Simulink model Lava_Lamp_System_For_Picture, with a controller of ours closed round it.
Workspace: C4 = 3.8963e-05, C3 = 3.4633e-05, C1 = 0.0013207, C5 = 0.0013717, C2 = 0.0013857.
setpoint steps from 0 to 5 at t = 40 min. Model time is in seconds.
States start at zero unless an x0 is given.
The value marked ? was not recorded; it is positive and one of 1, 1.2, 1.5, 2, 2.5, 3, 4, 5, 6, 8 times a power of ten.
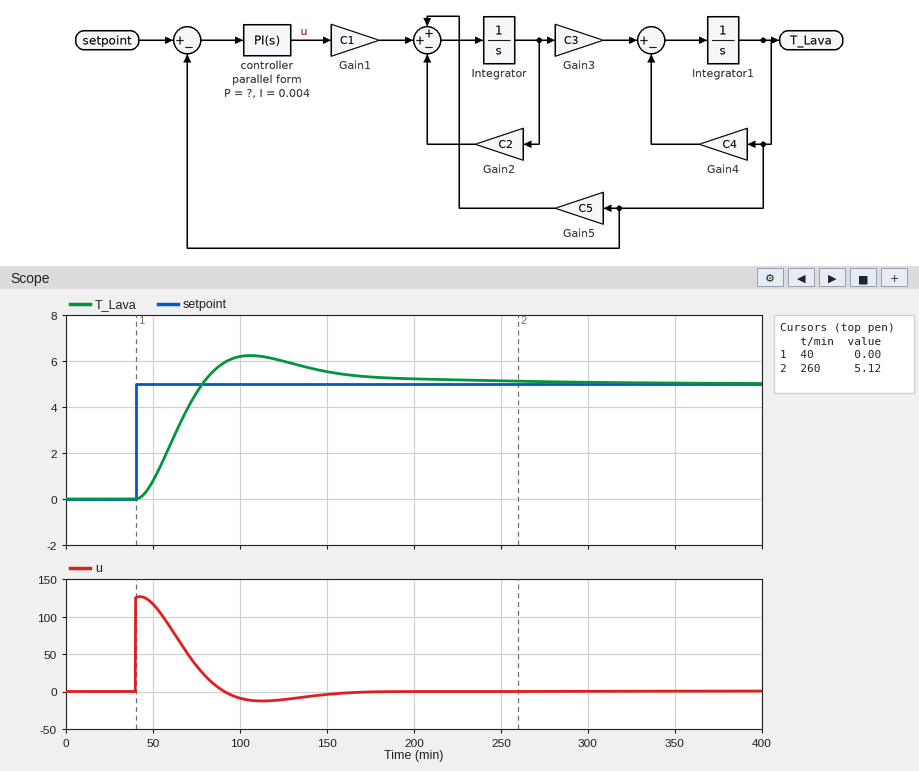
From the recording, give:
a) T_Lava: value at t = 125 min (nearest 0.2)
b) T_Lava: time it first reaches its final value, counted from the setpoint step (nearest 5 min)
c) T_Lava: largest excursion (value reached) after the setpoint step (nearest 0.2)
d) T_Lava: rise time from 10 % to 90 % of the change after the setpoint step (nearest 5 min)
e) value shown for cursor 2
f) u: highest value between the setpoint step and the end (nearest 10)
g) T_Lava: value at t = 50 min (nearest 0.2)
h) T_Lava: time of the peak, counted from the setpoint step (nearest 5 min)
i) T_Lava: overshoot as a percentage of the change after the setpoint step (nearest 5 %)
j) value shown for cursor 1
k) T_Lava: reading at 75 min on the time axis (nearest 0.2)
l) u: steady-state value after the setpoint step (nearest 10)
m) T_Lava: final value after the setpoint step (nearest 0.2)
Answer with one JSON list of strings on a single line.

["6.0", "40 min", "6.2", "25 min", "5.12", "130", "0.8", "65 min", "25 %", "0.00", "4.6", "0", "5.0"]
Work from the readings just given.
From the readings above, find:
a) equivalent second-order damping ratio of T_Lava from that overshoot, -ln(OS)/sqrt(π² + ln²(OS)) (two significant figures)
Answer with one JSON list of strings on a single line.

["0.40"]
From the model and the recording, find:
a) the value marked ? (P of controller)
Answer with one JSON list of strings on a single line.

["25"]
